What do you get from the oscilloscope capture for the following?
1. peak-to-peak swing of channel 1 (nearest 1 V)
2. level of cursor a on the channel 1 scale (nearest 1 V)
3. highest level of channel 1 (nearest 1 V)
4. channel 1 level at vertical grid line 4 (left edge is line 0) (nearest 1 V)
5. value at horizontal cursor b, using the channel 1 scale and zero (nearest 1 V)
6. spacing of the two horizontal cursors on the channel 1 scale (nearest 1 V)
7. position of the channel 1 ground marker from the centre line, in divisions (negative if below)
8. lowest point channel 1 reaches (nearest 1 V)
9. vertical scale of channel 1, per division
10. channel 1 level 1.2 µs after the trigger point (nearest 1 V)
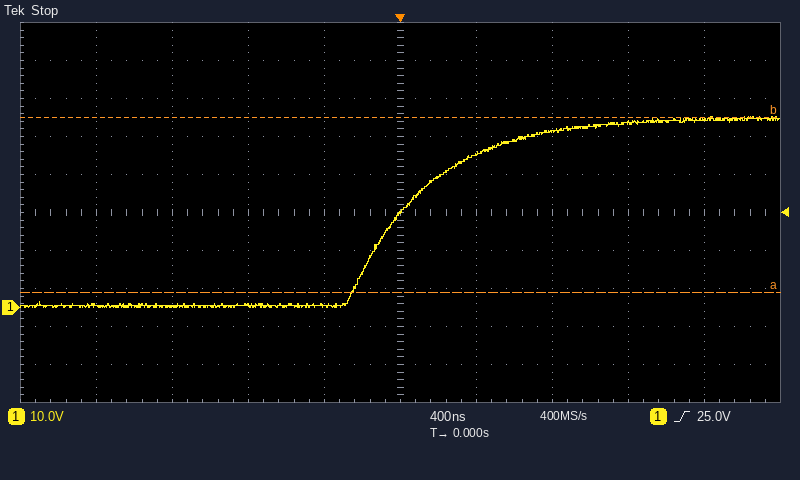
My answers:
50 V
4 V
50 V
1 V
50 V
46 V
-2.5 div
0 V
10 V
49 V
